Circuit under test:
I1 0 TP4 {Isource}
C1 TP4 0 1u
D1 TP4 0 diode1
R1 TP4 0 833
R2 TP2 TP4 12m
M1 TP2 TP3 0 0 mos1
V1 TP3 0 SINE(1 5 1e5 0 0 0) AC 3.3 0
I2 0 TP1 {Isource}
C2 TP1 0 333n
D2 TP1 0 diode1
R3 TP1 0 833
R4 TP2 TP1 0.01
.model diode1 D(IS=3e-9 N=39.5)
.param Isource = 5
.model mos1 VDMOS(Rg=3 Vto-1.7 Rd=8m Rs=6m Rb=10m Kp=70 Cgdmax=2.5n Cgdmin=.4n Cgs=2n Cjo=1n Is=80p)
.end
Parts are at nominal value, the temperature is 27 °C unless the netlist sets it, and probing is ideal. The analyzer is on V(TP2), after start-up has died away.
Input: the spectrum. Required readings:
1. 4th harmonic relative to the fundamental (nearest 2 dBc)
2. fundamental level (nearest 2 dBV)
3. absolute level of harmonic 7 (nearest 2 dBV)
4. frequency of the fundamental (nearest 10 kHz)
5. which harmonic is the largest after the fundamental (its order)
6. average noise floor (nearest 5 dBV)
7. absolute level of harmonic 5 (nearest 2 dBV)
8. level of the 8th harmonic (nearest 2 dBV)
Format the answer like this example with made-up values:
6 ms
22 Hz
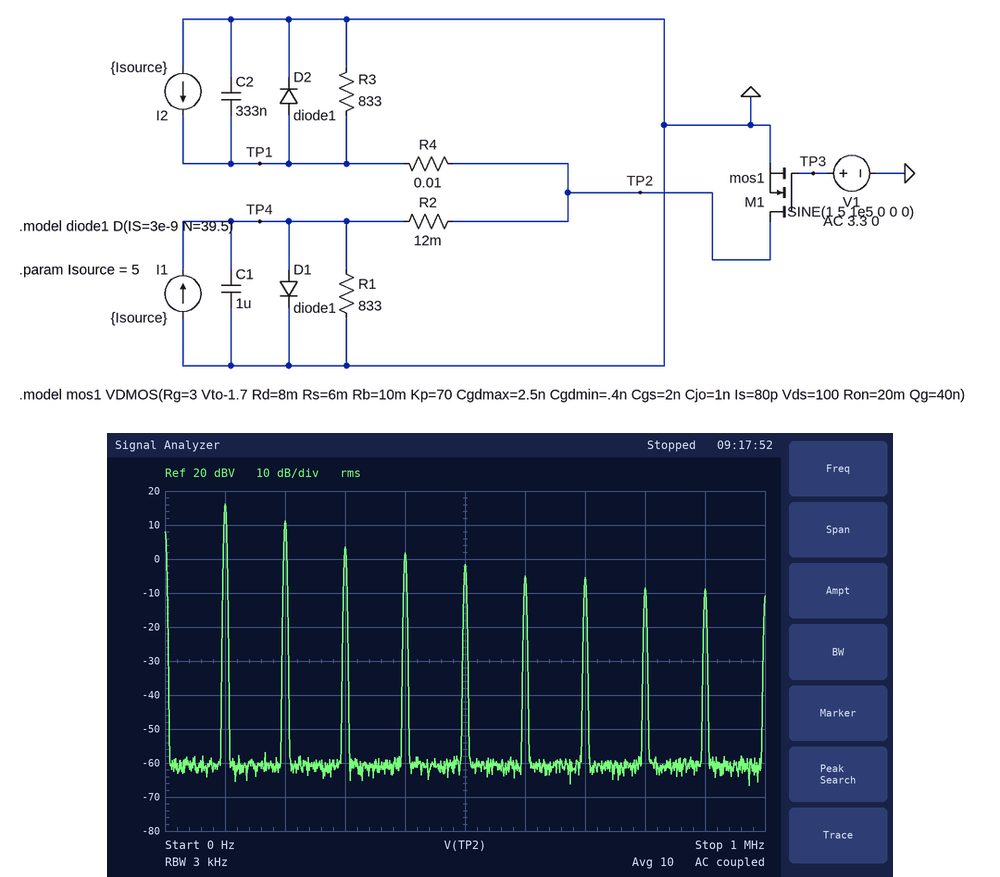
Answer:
-14 dBc
16 dBV
-6 dBV
100 kHz
2
-60 dBV
-2 dBV
-8 dBV
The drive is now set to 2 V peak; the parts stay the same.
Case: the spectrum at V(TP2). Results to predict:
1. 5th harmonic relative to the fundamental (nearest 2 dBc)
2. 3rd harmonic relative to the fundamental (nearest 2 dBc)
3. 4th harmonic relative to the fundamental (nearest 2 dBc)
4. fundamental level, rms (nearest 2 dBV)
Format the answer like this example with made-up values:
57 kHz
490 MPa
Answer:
-22 dBc
-12 dBc
-16 dBc
-24 dBV
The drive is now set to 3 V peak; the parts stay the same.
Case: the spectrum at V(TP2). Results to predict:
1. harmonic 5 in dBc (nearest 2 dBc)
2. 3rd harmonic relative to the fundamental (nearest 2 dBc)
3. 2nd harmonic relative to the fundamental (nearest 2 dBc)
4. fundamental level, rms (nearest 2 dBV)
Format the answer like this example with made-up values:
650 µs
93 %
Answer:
-16 dBc
-8 dBc
-2 dBc
12 dBV
